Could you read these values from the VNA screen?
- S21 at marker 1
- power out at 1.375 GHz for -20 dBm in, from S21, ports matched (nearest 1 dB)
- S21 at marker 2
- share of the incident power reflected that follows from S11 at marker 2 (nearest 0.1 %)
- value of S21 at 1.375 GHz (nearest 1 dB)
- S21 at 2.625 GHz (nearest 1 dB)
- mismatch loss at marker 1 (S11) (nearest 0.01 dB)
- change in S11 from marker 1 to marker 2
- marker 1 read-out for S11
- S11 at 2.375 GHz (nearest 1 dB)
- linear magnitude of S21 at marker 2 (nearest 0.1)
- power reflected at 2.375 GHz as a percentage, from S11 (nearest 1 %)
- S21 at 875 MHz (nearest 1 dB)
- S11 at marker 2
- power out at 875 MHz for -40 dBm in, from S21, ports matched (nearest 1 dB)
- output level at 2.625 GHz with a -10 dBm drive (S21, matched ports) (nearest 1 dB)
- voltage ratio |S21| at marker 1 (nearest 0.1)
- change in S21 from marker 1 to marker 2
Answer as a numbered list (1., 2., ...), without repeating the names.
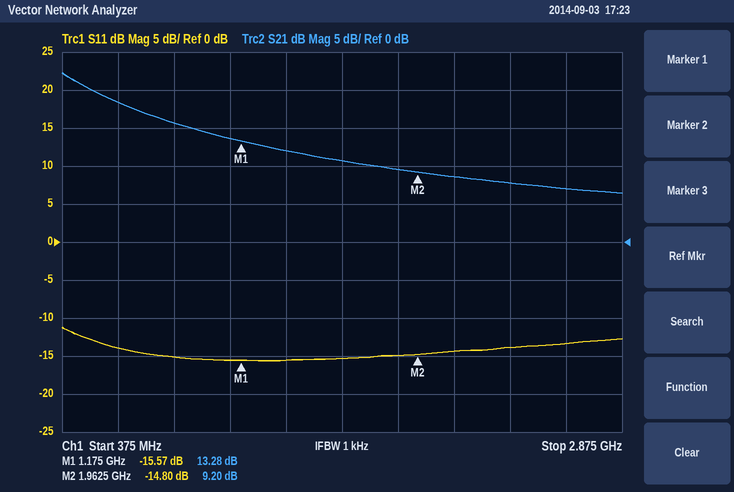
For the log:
1. 13.28 dB
2. -8 dBm
3. 9.20 dB
4. 3.3 %
5. 12 dB
6. 7 dB
7. 0.12 dB
8. 0.77 dB
9. -15.57 dB
10. -14 dB
11. 2.9
12. 4 %
13. 16 dB
14. -14.80 dB
15. -24 dBm
16. -3 dBm
17. 4.6
18. -4.08 dB
